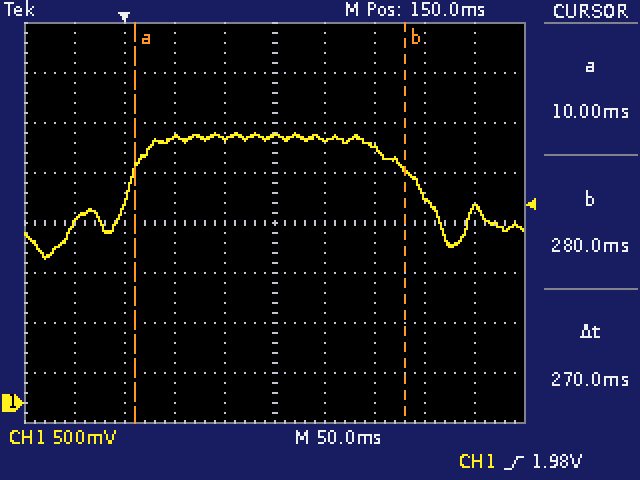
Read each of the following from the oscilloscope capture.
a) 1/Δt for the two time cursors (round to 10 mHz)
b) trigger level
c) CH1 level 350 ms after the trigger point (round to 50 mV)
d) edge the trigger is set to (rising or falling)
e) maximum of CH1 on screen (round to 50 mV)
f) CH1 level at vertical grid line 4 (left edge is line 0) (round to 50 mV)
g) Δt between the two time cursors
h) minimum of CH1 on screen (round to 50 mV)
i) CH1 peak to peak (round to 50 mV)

3.70 Hz
1.98 V
1.95 V
rising
2.70 V
2.65 V
270 ms
1.45 V
1.25 V
